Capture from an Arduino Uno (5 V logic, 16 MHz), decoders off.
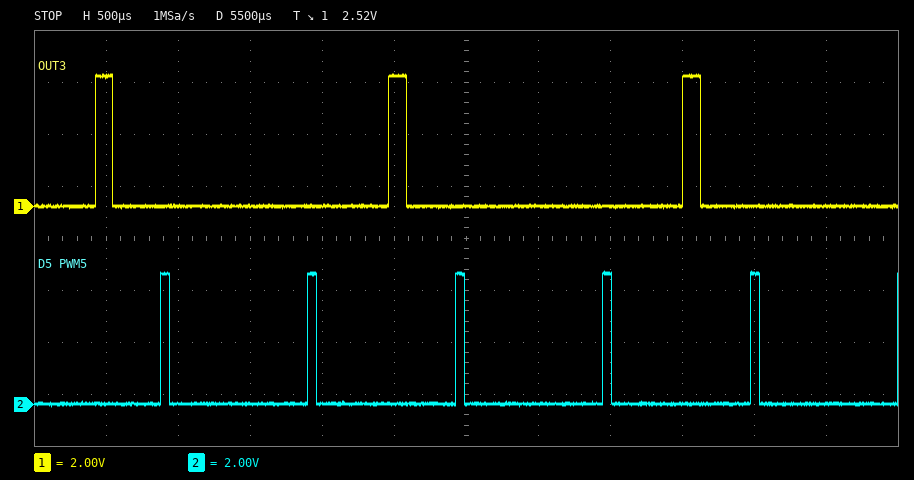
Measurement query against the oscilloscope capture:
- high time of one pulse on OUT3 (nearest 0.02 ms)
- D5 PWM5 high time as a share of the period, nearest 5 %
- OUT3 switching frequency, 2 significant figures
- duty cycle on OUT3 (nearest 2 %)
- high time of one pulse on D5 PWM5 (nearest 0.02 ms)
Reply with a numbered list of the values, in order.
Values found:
1. 0.12 ms
2. 5 %
3. 490 Hz
4. 6 %
5. 0.06 ms
